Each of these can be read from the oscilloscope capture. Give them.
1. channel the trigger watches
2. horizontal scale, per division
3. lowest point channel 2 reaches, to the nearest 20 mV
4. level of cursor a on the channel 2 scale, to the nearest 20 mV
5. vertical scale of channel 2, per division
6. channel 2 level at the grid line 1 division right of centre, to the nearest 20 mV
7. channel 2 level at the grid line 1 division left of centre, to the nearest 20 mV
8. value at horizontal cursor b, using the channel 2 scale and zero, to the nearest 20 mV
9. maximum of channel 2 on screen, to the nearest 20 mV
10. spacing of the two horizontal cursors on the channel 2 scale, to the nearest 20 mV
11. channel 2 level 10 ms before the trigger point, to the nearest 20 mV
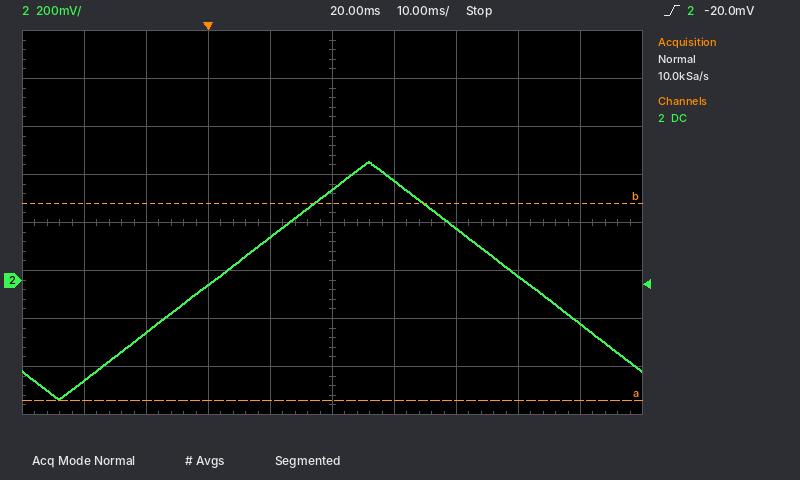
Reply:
channel 2
10 ms
-500 mV
-500 mV
200 mV
420 mV
180 mV
320 mV
500 mV
820 mV
-220 mV
